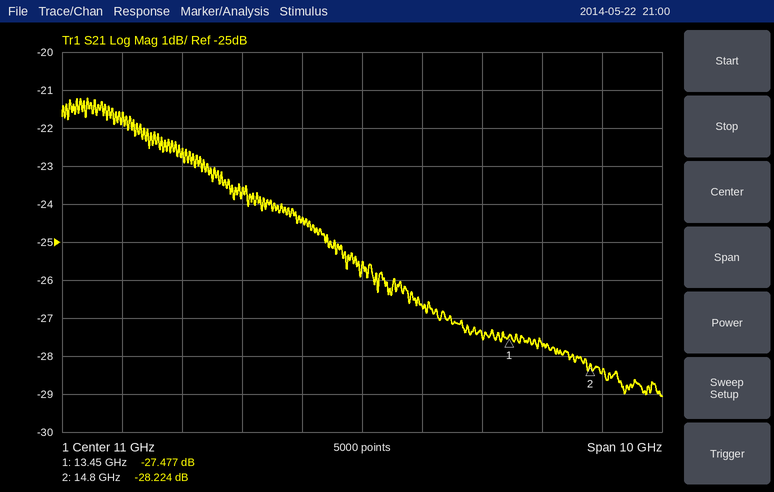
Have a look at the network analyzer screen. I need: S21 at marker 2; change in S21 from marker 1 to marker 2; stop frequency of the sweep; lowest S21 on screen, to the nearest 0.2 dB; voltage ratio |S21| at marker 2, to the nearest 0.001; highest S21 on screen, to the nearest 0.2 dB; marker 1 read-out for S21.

-28.224 dB
-0.747 dB
16 GHz
-29.0 dB
0.039
-21.2 dB
-27.477 dB
